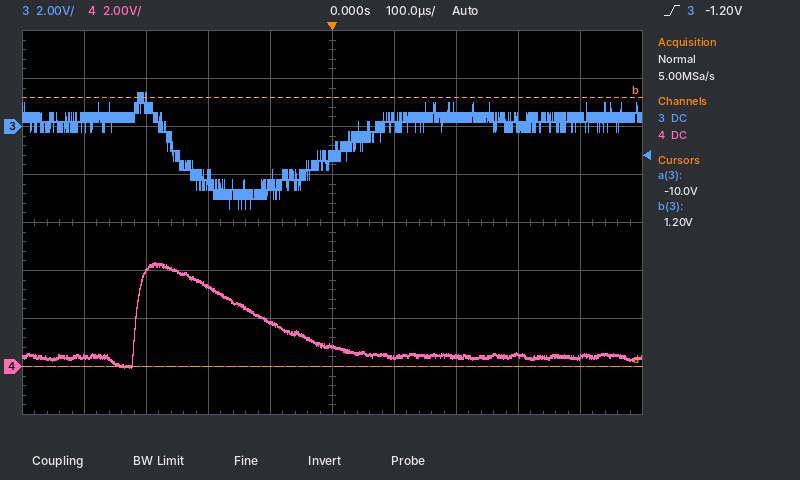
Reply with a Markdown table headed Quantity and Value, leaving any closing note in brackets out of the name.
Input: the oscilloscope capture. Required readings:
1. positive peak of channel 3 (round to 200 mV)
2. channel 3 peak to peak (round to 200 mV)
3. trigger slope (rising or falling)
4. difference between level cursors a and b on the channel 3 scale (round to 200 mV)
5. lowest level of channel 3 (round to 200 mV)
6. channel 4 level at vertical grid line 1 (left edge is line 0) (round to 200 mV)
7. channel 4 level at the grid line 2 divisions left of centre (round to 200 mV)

| Quantity | Value |
|---|---|
| positive peak of channel 3 | 1.4 V |
| channel 3 peak to peak | 4.8 V |
| trigger slope | rising |
| difference between level cursors a and b on the channel 3 scale | 11.2 V |
| lowest level of channel 3 | -3.4 V |
| channel 4 level at vertical grid line 1 (left edge is line 0) | 400 mV |
| channel 4 level at the grid line 2 divisions left of centre | 3.4 V |
